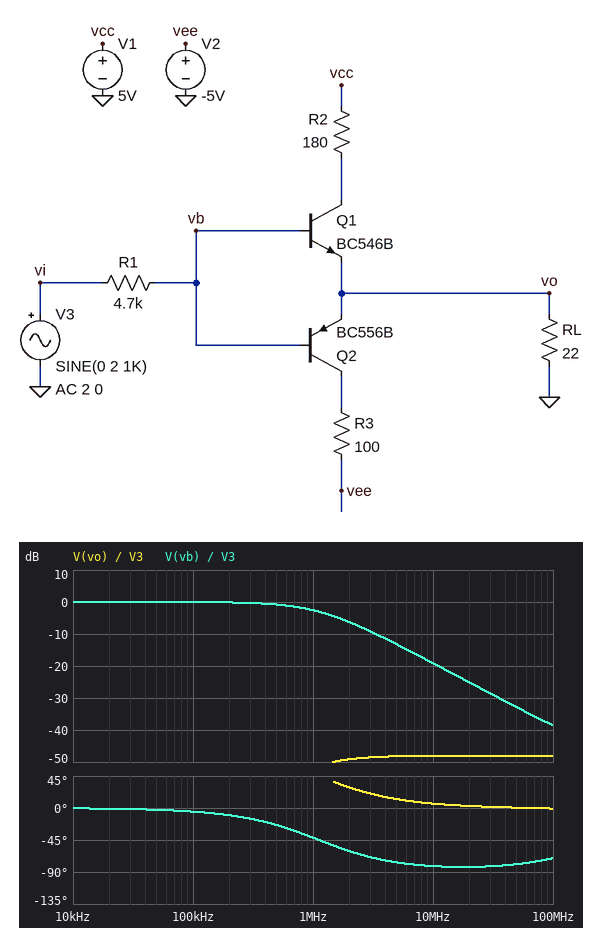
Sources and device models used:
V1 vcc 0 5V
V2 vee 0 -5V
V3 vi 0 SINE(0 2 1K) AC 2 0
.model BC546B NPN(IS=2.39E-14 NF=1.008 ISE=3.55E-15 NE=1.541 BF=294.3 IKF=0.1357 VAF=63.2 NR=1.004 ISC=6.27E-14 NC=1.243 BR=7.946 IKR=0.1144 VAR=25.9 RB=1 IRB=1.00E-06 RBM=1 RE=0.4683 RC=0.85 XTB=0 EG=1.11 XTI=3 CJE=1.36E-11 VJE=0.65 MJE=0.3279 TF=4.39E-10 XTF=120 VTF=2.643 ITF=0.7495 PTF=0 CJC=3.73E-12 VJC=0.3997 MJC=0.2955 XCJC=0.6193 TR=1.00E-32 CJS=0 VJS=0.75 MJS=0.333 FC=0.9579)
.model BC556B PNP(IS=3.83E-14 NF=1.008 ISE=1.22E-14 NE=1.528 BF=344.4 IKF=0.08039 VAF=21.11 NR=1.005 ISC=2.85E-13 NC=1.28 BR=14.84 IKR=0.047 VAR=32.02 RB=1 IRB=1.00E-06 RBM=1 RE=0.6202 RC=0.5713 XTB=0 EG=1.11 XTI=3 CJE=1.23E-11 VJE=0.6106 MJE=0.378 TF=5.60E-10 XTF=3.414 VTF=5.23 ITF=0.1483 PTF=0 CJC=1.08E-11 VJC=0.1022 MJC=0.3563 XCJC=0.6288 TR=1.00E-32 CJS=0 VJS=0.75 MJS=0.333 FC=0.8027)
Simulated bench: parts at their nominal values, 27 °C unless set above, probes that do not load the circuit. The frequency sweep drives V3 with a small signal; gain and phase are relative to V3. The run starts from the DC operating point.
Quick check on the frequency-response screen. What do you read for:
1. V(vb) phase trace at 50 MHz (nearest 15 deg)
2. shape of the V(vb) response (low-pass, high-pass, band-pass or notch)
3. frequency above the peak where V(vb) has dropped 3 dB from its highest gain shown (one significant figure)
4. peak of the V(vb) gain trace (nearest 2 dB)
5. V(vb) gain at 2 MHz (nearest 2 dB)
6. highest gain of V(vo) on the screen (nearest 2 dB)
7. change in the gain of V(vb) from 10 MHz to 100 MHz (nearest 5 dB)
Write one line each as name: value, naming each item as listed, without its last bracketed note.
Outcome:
V(vb) phase trace at 50 MHz: -75 deg
shape of the V(vb) response: low-pass
frequency above the peak where V(vb) has dropped 3 dB from its highest gain shown: 1 MHz
peak of the V(vb) gain trace: 0 dB
V(vb) gain at 2 MHz: -6 dB
highest gain of V(vo) on the screen: -48 dB
change in the gain of V(vb) from 10 MHz to 100 MHz: -20 dB
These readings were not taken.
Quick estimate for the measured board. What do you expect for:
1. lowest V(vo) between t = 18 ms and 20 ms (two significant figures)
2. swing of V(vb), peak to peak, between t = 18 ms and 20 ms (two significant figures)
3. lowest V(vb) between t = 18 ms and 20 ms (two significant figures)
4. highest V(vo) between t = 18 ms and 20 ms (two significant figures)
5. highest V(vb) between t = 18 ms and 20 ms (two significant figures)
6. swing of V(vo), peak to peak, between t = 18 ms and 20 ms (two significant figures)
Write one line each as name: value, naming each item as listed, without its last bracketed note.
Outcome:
lowest V(vo) between t = 18 ms and 20 ms: -680 mV
swing of V(vb), peak to peak, between t = 18 ms and 20 ms: 2.7 V
lowest V(vb) between t = 18 ms and 20 ms: -1.4 V
highest V(vo) between t = 18 ms and 20 ms: 530 mV
highest V(vb) between t = 18 ms and 20 ms: 1.3 V
swing of V(vo), peak to peak, between t = 18 ms and 20 ms: 1.2 V
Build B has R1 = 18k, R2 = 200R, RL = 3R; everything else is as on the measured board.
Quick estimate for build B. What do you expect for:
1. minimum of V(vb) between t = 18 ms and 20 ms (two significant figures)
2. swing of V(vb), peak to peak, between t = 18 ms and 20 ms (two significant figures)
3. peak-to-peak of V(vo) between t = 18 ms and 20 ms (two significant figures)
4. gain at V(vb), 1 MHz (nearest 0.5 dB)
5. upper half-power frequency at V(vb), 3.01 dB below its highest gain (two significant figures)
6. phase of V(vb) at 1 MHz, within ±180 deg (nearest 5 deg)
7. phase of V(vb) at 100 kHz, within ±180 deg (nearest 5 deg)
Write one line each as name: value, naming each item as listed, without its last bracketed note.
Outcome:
minimum of V(vb) between t = 18 ms and 20 ms: -780 mV
swing of V(vb), peak to peak, between t = 18 ms and 20 ms: 1.6 V
peak-to-peak of V(vo) between t = 18 ms and 20 ms: 110 mV
gain at V(vb), 1 MHz: -11.0 dB
upper half-power frequency at V(vb), 3.01 dB below its highest gain: 290 kHz
phase of V(vb) at 1 MHz, within ±180 deg: -75 deg
phase of V(vb) at 100 kHz, within ±180 deg: -20 deg
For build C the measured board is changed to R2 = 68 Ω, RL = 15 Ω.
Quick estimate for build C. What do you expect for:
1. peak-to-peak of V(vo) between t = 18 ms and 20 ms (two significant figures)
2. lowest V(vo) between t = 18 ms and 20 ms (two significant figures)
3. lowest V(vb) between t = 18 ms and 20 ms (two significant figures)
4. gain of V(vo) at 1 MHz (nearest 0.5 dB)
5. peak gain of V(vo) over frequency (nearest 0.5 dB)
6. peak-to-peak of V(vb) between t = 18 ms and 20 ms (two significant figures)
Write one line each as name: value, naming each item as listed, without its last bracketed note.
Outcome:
peak-to-peak of V(vo) between t = 18 ms and 20 ms: 1.1 V
lowest V(vo) between t = 18 ms and 20 ms: -530 mV
lowest V(vb) between t = 18 ms and 20 ms: -1.3 V
gain of V(vo) at 1 MHz: -55.0 dB
peak gain of V(vo) over frequency: -51.5 dB
peak-to-peak of V(vb) between t = 18 ms and 20 ms: 2.6 V
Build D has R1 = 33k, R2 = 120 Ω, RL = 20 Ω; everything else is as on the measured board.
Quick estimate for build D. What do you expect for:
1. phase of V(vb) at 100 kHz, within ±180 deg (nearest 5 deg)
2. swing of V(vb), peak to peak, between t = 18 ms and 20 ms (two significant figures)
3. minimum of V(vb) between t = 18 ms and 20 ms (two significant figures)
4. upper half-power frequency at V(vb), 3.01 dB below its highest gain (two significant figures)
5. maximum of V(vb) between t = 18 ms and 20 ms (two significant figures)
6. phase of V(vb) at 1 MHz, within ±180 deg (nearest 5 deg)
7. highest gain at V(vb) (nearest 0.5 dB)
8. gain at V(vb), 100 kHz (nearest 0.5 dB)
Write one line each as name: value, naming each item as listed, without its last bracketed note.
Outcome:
phase of V(vb) at 100 kHz, within ±180 deg: -30 deg
swing of V(vb), peak to peak, between t = 18 ms and 20 ms: 1.8 V
minimum of V(vb) between t = 18 ms and 20 ms: -920 mV
upper half-power frequency at V(vb), 3.01 dB below its highest gain: 160 kHz
maximum of V(vb) between t = 18 ms and 20 ms: 890 mV
phase of V(vb) at 1 MHz, within ±180 deg: -80 deg
highest gain at V(vb): 0 dB
gain at V(vb), 100 kHz: -1.5 dB
